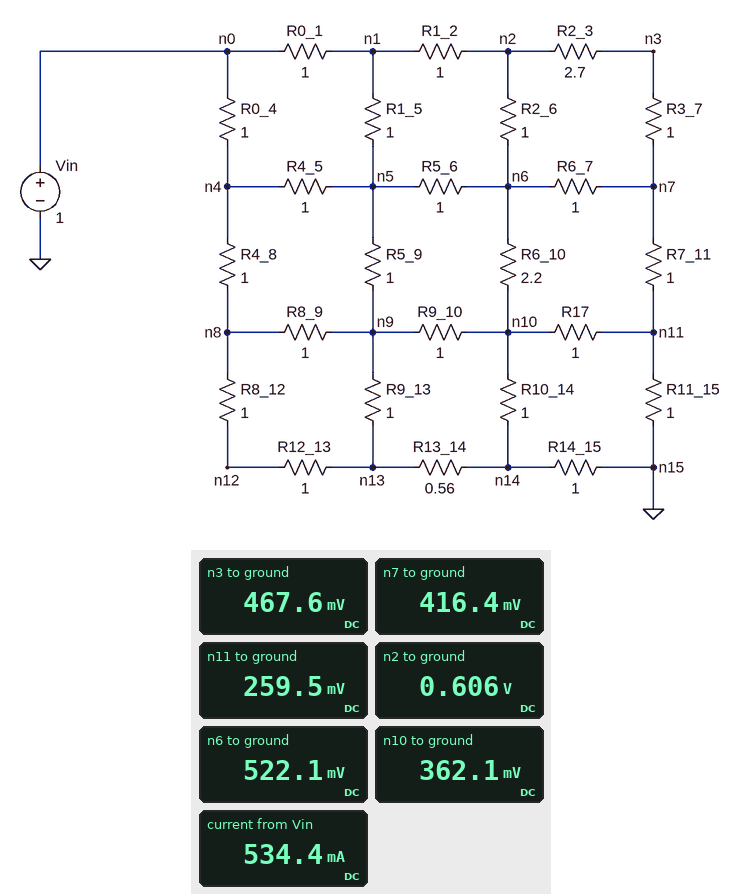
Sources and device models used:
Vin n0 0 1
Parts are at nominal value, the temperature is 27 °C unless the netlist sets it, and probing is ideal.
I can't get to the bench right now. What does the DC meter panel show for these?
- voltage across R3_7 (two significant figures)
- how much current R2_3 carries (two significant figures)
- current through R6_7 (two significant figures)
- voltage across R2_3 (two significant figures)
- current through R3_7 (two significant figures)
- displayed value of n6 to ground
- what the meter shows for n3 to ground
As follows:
51 mV
51 mA
110 mA
140 mV
51 mA
522.1 mV
467.6 mV
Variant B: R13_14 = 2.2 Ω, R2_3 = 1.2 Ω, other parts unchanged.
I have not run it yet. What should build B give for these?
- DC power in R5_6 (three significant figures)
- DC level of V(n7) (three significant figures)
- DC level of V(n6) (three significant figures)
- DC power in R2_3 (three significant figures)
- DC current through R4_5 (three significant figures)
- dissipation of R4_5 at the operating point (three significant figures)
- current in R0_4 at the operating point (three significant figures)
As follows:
10.5 mW
439 mV
535 mV
6.69 mW
109 mA
11.9 mW
254 mA
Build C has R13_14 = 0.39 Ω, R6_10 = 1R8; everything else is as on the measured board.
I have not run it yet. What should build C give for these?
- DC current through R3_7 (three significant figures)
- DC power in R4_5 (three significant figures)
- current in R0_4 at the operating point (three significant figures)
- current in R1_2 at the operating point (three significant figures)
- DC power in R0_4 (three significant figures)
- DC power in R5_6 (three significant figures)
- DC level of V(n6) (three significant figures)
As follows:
50.8 mA
12.0 mW
280 mA
137 mA
78.4 mW
9.46 mW
513 mV
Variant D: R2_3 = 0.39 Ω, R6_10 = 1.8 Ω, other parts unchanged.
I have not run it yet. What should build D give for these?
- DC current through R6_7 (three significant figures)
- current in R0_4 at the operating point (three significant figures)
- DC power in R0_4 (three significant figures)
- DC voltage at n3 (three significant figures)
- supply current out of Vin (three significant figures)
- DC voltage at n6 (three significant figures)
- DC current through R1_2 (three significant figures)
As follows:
74.6 mA
277 mA
76.6 mW
537 mV
548 mA
515 mV
155 mA
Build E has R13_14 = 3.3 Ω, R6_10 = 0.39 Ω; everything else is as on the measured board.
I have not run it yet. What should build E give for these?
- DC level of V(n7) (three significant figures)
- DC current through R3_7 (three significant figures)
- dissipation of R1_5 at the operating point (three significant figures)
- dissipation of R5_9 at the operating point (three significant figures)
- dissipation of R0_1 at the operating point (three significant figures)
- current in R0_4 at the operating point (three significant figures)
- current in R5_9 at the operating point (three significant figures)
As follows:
399 mV
49.6 mA
12.1 mW
7.03 mW
69.6 mW
252 mA
83.9 mA
